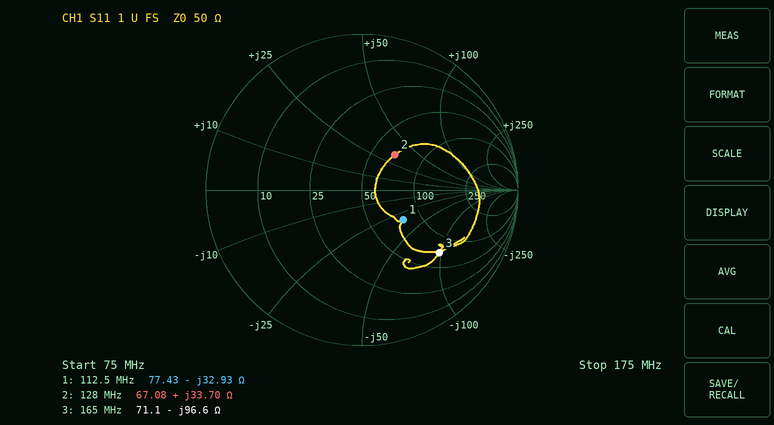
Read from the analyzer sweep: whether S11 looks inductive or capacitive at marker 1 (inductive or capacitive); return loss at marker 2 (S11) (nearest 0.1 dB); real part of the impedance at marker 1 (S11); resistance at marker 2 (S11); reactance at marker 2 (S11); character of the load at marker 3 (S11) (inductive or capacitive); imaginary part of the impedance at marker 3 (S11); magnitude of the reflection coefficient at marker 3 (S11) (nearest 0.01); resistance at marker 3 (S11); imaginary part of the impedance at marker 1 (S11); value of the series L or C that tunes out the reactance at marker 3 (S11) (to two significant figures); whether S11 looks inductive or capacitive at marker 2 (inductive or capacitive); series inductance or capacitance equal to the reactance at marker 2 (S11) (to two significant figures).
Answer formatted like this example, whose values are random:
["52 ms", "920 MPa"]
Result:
["capacitive", "10.2 dB", "77.43 Ω", "67.08 Ω", "+33.70 Ω", "capacitive", "-96.6 Ω", "0.64", "71.1 Ω", "-32.93 Ω", "93 nH", "inductive", "42 nH"]
